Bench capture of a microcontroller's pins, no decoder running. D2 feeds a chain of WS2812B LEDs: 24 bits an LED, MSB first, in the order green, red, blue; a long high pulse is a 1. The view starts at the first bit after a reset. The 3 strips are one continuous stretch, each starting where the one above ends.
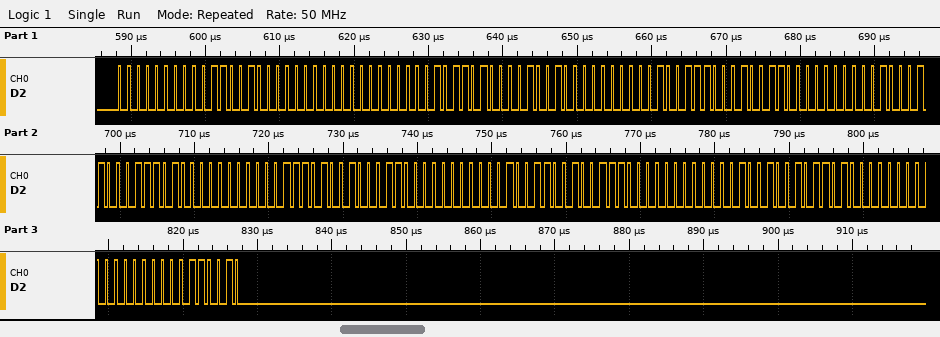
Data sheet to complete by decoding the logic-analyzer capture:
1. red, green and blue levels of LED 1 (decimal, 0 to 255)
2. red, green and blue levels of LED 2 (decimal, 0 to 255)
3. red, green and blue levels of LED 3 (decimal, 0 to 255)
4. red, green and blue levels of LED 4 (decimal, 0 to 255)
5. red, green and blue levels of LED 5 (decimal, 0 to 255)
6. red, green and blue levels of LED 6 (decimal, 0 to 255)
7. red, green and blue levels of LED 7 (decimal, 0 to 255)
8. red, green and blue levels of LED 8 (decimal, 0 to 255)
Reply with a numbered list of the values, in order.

1. 50, 0, 0
2. 45, 0, 9
3. 39, 0, 19
4. 35, 0, 29
5. 29, 0, 35
6. 19, 0, 39
7. 9, 0, 45
8. 0, 0, 50
